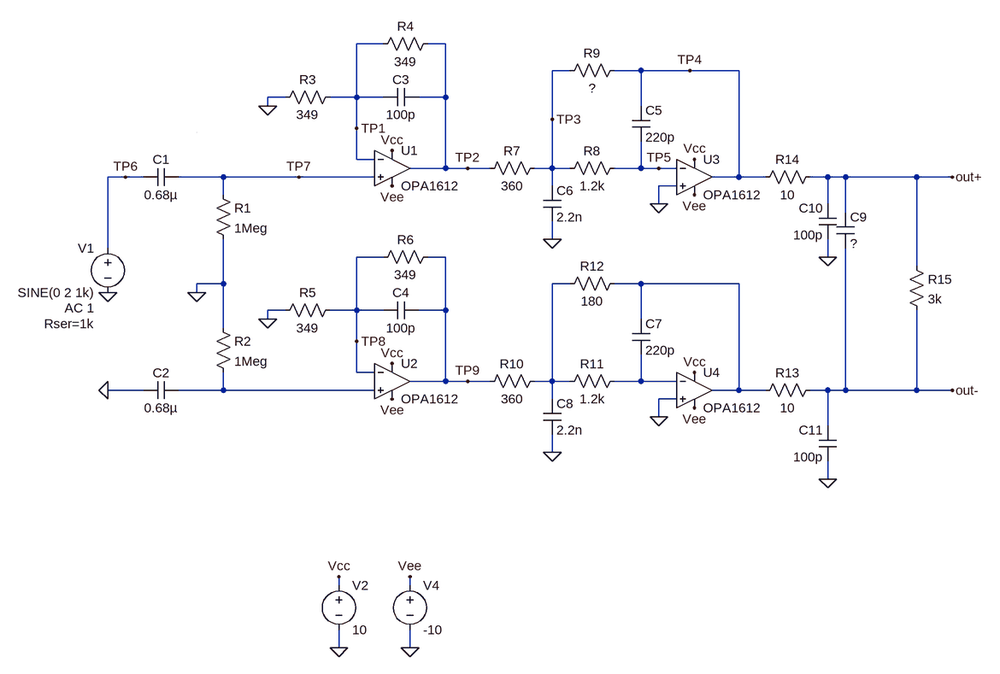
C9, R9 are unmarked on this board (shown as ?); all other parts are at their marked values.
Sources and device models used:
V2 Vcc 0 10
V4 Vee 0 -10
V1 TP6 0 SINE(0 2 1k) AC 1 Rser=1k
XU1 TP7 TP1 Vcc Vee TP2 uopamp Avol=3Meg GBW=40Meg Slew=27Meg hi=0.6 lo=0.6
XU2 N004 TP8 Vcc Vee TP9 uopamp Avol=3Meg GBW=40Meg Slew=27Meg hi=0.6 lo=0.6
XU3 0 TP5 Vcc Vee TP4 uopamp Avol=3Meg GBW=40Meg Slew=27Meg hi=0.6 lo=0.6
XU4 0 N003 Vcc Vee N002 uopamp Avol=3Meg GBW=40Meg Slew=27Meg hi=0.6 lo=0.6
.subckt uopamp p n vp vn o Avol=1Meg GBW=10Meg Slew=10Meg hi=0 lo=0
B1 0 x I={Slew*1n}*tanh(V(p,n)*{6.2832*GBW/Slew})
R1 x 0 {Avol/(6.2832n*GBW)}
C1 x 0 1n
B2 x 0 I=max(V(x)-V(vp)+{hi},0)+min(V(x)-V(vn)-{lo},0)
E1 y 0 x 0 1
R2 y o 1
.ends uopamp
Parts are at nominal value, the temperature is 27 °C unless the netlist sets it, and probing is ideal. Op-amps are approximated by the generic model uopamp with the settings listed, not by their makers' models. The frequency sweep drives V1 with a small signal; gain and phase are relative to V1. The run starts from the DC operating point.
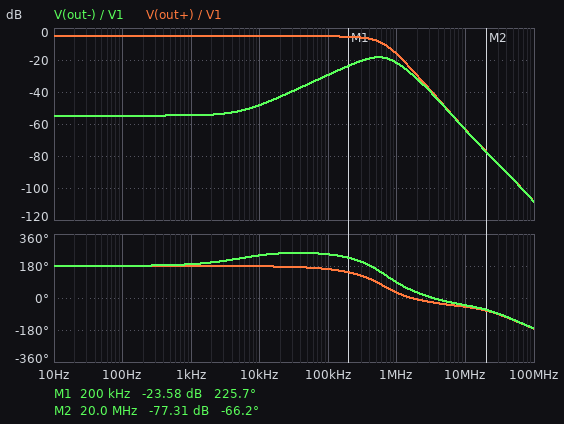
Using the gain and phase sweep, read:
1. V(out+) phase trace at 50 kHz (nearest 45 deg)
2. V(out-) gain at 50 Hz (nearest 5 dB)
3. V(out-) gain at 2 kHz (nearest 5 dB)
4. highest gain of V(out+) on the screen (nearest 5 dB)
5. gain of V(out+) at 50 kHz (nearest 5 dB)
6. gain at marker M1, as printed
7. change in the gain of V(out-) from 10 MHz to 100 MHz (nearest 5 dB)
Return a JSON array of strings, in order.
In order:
["180 deg", "-55 dB", "-55 dB", "-5 dB", "-5 dB", "-23.58 dB", "-45 dB"]
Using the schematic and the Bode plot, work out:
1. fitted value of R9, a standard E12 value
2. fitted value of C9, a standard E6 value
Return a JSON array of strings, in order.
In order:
["100 Ω", "10 nF"]
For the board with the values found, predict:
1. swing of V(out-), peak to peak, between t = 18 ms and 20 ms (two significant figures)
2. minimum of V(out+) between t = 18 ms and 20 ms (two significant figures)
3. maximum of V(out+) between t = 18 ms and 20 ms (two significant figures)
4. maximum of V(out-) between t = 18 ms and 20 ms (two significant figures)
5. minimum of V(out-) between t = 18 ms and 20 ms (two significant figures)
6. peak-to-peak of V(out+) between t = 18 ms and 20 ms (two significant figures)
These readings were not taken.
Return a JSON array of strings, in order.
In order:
["7.5 mV", "-1.1 V", "1.1 V", "3.7 mV", "-3.7 mV", "2.2 V"]
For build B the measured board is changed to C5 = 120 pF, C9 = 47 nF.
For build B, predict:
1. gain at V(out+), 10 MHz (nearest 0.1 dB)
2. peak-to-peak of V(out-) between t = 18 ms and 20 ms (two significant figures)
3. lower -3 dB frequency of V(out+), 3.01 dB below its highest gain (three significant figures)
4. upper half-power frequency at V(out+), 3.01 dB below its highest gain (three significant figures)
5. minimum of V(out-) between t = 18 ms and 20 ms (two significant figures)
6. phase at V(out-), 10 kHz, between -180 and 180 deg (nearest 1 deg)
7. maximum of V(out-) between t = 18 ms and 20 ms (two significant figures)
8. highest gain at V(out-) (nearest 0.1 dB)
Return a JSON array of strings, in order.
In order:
["-58.6 dB", "9.8 mV", "234 mHz", "266 kHz", "-4.9 mV", "-101 deg", "4.9 mV", "-10.8 dB"]
